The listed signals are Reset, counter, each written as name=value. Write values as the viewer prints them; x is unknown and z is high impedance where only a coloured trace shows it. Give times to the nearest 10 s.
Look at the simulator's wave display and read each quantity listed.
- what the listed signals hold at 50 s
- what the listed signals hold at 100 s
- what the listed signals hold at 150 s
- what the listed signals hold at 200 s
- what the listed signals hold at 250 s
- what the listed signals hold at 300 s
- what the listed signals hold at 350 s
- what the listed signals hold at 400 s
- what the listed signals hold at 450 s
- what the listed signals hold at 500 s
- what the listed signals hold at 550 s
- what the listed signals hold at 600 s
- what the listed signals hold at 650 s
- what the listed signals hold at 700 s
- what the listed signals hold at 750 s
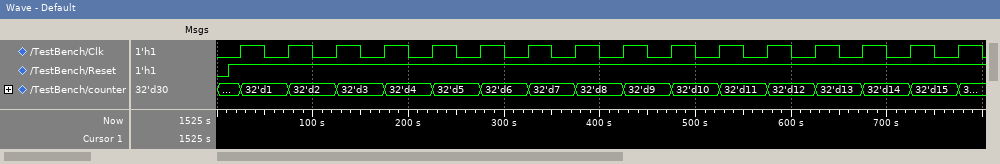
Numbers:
Reset=1, counter=32'd1
Reset=1, counter=32'd2
Reset=1, counter=32'd3
Reset=1, counter=32'd4
Reset=1, counter=32'd5
Reset=1, counter=32'd6
Reset=1, counter=32'd7
Reset=1, counter=32'd8
Reset=1, counter=32'd9
Reset=1, counter=32'd10
Reset=1, counter=32'd11
Reset=1, counter=32'd12
Reset=1, counter=32'd13
Reset=1, counter=32'd14
Reset=1, counter=32'd15
